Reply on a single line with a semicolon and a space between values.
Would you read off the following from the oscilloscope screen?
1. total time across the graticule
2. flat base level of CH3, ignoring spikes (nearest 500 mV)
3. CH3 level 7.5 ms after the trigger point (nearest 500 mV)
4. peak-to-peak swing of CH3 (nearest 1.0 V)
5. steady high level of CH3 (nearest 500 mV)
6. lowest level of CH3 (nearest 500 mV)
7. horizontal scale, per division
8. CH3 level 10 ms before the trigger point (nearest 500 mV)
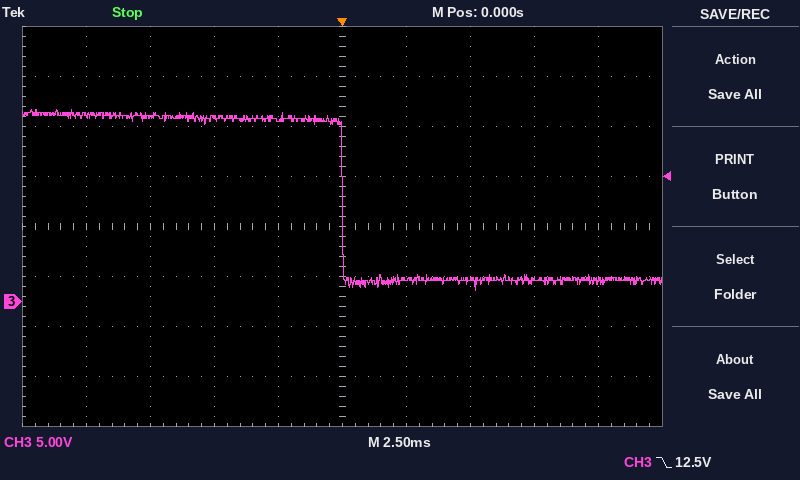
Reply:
25 ms; 2.0 V; 2.0 V; 18.0 V; 18.5 V; 1.0 V; 2.5 ms; 18.5 V
